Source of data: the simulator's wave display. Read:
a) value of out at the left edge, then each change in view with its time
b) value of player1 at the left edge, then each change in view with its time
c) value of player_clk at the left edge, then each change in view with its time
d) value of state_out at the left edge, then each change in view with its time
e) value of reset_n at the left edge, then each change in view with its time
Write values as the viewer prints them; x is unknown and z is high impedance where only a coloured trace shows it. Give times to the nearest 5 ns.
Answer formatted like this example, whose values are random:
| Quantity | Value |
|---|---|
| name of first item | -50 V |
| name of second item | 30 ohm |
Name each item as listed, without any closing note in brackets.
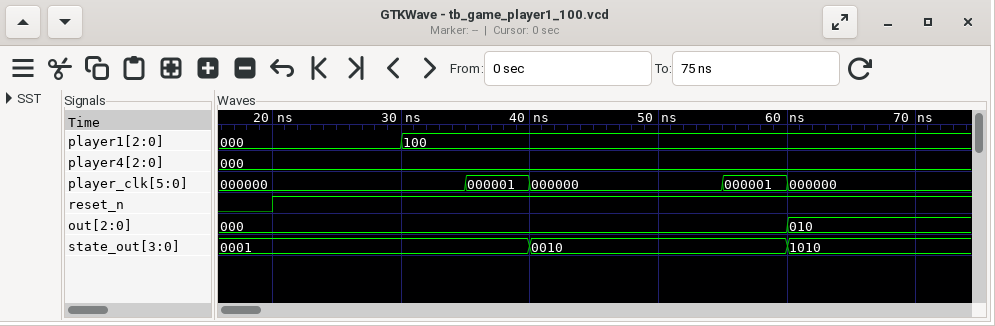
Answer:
| Quantity | Value |
|---|---|
| value of out at the left edge, then each change in view with its time | 000, 010 at 60 ns |
| value of player1 at the left edge, then each change in view with its time | 000, 100 at 30 ns |
| value of player_clk at the left edge, then each change in view with its time | 000000, 000001 at 35 ns, 000000 at 40 ns, 000001 at 55 ns, 000000 at 60 ns |
| value of state_out at the left edge, then each change in view with its time | 0001, 0010 at 40 ns, 1010 at 60 ns |
| value of reset_n at the left edge, then each change in view with its time | 0, 1 at 20 ns |
